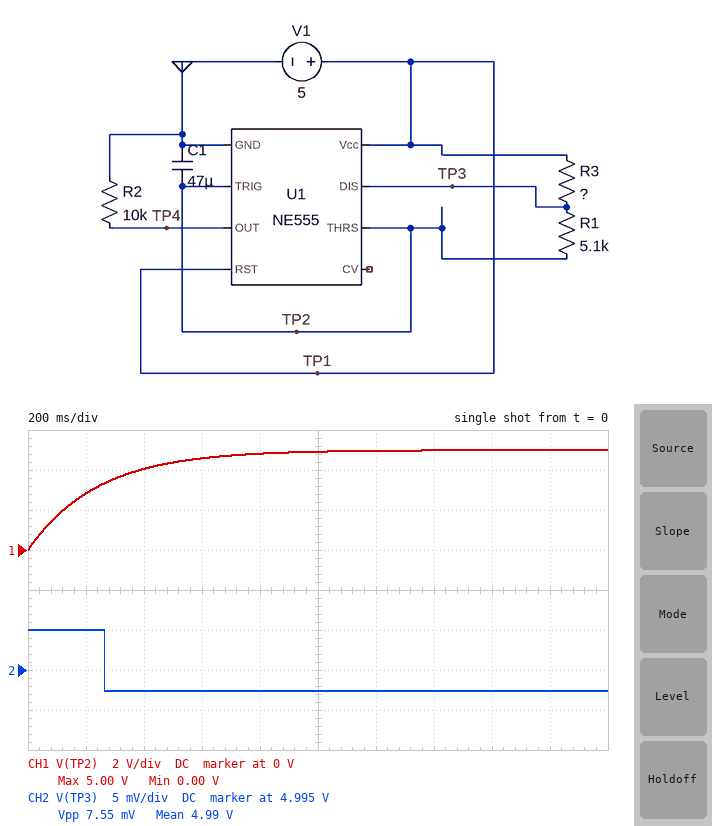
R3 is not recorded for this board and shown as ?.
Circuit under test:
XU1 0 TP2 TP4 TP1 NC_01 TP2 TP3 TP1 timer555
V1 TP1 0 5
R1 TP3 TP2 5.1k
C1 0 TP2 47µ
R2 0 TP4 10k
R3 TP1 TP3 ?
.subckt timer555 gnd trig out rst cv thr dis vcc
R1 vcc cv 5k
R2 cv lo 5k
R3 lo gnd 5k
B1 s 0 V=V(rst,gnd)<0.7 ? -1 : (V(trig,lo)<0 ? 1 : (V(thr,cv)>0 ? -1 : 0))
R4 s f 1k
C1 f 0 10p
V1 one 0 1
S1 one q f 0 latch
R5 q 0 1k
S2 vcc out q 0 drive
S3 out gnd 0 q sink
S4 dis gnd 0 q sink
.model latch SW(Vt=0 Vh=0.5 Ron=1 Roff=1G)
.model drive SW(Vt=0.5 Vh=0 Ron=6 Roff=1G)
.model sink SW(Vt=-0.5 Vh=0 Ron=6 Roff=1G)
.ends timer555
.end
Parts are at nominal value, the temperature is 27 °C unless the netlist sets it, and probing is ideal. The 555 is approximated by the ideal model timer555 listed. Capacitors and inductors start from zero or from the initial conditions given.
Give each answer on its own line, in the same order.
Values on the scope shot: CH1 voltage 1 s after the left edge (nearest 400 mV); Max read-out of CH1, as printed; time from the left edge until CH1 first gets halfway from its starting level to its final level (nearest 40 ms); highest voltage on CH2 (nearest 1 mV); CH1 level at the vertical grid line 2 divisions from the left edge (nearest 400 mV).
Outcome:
4.8 V
5.00 V
160 ms
5.000 V
4.0 V
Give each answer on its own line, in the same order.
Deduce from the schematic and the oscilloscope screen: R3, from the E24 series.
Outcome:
9.1 mΩ
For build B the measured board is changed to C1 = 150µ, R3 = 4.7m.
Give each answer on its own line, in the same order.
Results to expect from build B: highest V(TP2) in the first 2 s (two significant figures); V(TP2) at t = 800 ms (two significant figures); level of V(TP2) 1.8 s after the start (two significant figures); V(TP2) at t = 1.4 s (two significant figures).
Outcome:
4.6 V
3.2 V
4.5 V
4.2 V
